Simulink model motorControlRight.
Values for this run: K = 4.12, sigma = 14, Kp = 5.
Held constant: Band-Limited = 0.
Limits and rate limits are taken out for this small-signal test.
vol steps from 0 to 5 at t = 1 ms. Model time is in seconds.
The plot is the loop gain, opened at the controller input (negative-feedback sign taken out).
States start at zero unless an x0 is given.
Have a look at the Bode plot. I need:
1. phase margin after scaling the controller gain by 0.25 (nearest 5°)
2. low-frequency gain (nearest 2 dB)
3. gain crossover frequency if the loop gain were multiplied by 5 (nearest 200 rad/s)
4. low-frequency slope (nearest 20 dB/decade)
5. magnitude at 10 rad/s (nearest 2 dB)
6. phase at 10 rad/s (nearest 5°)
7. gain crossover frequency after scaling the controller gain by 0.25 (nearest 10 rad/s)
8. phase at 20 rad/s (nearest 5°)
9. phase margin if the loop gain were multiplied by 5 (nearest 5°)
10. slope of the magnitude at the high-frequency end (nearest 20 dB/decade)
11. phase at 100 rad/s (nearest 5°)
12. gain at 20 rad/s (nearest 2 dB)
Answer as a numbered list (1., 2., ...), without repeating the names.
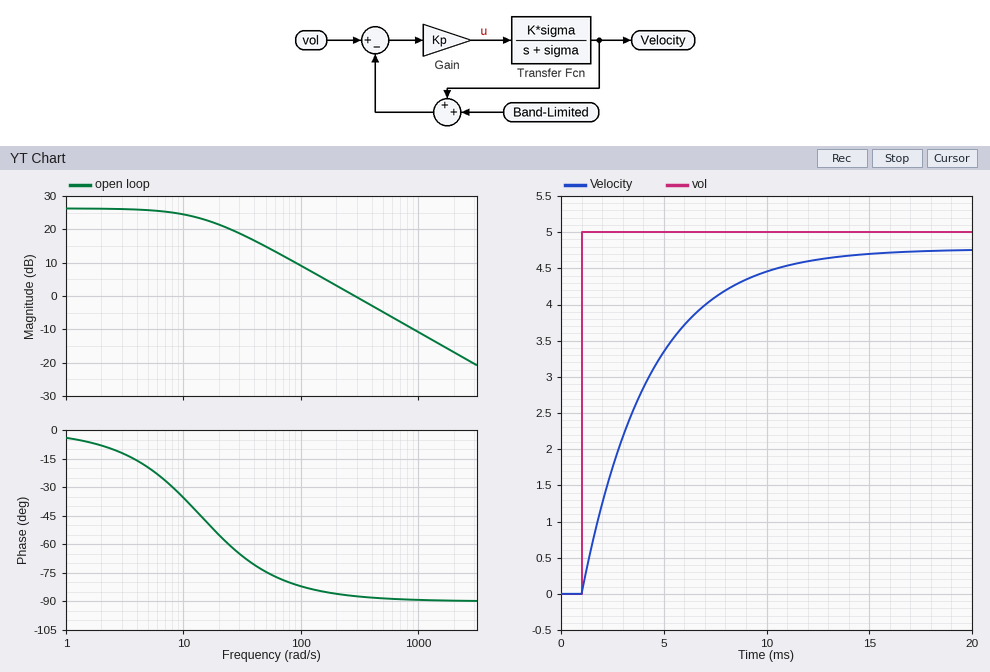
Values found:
1. 100°
2. 26 dB
3. 1400 rad/s
4. 0 dB/decade
5. 24 dB
6. -35°
7. 70 rad/s
8. -55°
9. 90°
10. -20 dB/decade
11. -80°
12. 22 dB
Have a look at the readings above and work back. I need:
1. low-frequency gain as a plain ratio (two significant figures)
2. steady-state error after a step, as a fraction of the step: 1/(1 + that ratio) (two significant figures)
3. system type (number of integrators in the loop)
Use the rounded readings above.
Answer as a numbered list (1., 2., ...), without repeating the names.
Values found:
1. 20
2. 0.048
3. 0
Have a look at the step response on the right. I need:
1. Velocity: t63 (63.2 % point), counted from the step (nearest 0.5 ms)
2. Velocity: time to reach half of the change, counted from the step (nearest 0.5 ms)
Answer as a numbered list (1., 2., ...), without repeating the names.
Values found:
1. 3.5 ms
2. 2.5 ms
